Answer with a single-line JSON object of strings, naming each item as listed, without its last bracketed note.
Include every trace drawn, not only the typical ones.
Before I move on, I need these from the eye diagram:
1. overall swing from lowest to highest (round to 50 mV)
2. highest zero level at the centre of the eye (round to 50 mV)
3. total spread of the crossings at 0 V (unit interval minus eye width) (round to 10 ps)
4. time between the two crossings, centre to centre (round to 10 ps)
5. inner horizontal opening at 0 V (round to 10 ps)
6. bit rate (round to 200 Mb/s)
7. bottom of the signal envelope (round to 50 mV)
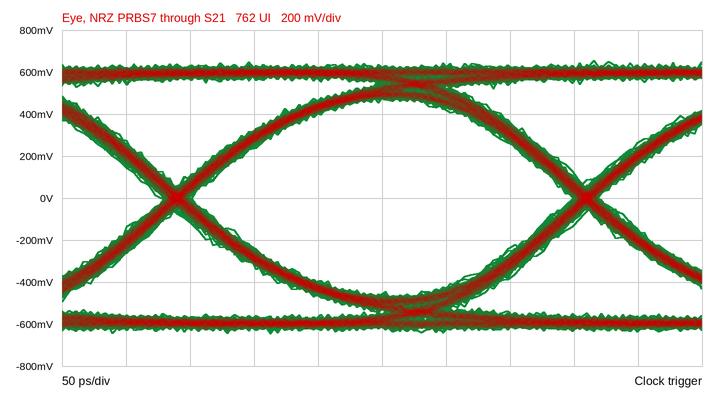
{"overall swing from lowest to highest": "1.30 V", "highest zero level at the centre of the eye": "-450 mV", "total spread of the crossings at 0 V (unit interval minus eye width)": "20 ps", "time between the two crossings, centre to centre": "320 ps", "inner horizontal opening at 0 V": "300 ps", "bit rate": "3.2 Gb/s", "bottom of the signal envelope": "-650 mV"}
